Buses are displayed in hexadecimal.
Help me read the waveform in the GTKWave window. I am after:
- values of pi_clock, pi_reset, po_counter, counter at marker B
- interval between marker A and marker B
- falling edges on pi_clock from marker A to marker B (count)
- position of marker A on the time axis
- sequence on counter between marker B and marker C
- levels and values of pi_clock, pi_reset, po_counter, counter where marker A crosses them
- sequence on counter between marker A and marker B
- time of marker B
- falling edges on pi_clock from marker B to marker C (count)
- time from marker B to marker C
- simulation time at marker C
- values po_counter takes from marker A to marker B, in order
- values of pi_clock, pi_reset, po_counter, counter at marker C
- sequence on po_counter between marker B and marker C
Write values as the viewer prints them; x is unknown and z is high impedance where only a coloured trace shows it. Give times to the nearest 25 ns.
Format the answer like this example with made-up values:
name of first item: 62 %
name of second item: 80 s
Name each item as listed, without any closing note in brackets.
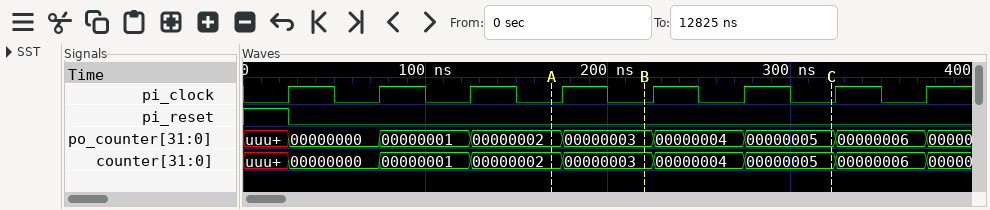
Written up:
values of pi_clock, pi_reset, po_counter, counter at marker B: pi_clock=0, pi_reset=0, po_counter=00000003, counter=00000003
interval between marker A and marker B: 50 ns
falling edges on pi_clock from marker A to marker B: 1
position of marker A on the time axis: 175 ns
sequence on counter between marker B and marker C: 00000003, 00000004, 00000005
levels and values of pi_clock, pi_reset, po_counter, counter where marker A crosses them: pi_clock=0, pi_reset=0, po_counter=00000002, counter=00000002
sequence on counter between marker A and marker B: 00000002, 00000003
time of marker B: 225 ns
falling edges on pi_clock from marker B to marker C: 2
time from marker B to marker C: 100 ns
simulation time at marker C: 325 ns
values po_counter takes from marker A to marker B, in order: 00000002, 00000003
values of pi_clock, pi_reset, po_counter, counter at marker C: pi_clock=0, pi_reset=0, po_counter=00000005, counter=00000005
sequence on po_counter between marker B and marker C: 00000003, 00000004, 00000005
